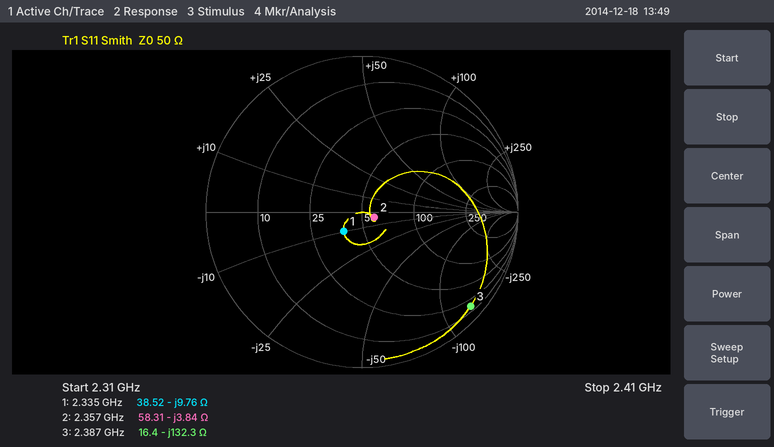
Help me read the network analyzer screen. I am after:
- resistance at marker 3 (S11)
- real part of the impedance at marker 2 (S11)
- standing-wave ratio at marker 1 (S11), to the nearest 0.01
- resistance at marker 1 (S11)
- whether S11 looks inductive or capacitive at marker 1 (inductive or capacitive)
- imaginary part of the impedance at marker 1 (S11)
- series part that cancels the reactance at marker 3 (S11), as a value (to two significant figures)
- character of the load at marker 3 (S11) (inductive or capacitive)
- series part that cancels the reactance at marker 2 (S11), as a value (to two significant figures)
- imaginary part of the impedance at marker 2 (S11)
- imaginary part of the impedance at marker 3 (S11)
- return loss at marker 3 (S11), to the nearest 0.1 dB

16.4 Ω
58.31 Ω
1.41
38.52 Ω
capacitive
-9.76 Ω
8.8 nH
capacitive
260 pH
-3.84 Ω
-132.3 Ω
0.7 dB
